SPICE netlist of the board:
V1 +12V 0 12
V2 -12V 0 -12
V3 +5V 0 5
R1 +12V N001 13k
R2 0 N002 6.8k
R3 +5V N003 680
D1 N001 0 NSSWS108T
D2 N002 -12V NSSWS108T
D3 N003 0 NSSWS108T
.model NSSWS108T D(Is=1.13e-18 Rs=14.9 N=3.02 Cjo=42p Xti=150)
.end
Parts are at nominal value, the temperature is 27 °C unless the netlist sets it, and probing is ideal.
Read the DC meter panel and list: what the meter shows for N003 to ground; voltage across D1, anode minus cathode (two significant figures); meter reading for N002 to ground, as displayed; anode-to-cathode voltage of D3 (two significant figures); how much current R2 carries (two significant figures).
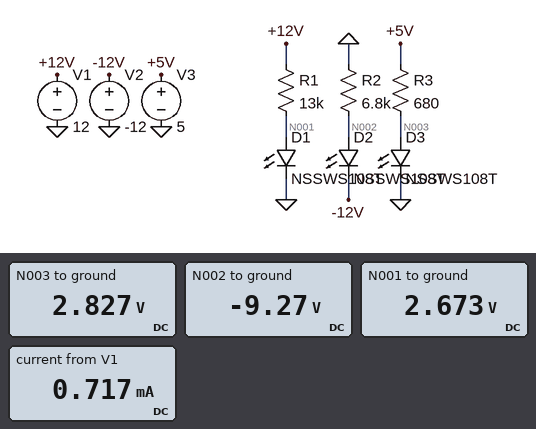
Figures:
2.827 V
2.7 V
-9.27 V
2.8 V
1.4 mA
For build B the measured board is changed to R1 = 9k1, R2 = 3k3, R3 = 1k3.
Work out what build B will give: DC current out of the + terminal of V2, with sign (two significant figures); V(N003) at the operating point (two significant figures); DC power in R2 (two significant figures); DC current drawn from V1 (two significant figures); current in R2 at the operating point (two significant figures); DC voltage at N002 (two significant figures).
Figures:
-2.8 mA
2.8 V
26 mW
1.0 mA
2.8 mA
-9.2 V
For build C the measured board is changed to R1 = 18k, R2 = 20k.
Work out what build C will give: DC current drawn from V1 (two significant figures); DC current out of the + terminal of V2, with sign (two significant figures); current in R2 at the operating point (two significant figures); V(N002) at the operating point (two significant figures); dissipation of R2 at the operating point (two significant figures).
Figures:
520 µA
-470 µA
470 µA
-9.4 V
4.4 mW
